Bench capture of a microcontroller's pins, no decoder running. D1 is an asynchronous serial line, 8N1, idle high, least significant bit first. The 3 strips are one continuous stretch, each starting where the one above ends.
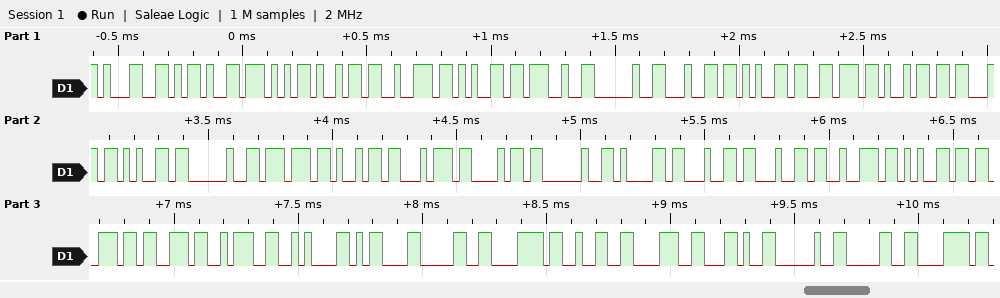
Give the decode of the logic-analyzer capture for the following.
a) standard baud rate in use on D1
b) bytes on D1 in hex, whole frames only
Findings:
38400 baud
0x31 0x2D 0x57 0x69 0x72 0x65 0x27 0x20 0x64 0x65 0x76 0x69 0x63 0x65 0x20 0x77 0x69 0x74 0x68 0x20 0x61 0x64 0x64 0x72 0x65 0x73 0x73 0x3A 0x0A 0x0D 0x30 0x78 0x32 0x38 0x2C 0x20 0x30 0x78
